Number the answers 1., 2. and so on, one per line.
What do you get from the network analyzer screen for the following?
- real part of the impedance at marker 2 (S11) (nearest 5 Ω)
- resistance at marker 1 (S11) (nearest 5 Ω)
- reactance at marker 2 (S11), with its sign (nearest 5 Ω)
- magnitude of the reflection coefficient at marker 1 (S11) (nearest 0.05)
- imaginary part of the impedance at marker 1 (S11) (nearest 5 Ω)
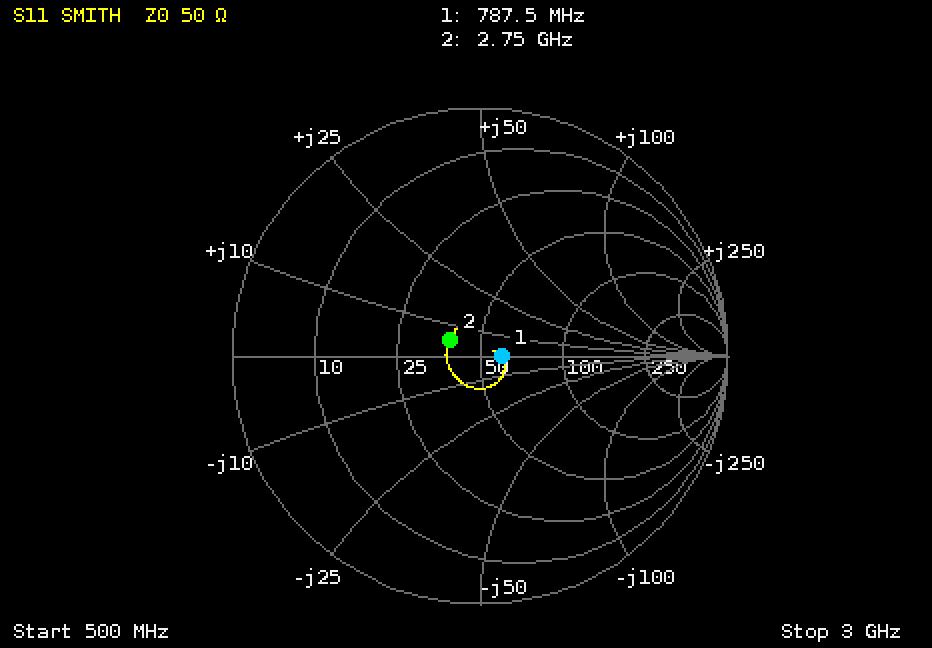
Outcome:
1. 40 Ω
2. 60 Ω
3. +5 Ω
4. 0.10
5. 0 Ω
